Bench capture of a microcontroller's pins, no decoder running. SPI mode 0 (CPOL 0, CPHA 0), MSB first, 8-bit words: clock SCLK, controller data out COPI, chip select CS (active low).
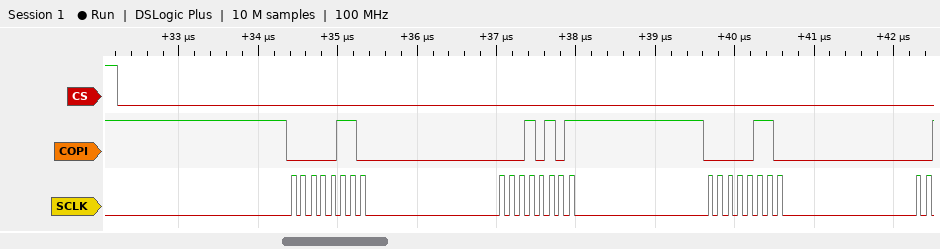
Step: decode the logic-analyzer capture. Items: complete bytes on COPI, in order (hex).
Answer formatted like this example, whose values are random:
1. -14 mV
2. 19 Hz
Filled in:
1. 06 15 06
